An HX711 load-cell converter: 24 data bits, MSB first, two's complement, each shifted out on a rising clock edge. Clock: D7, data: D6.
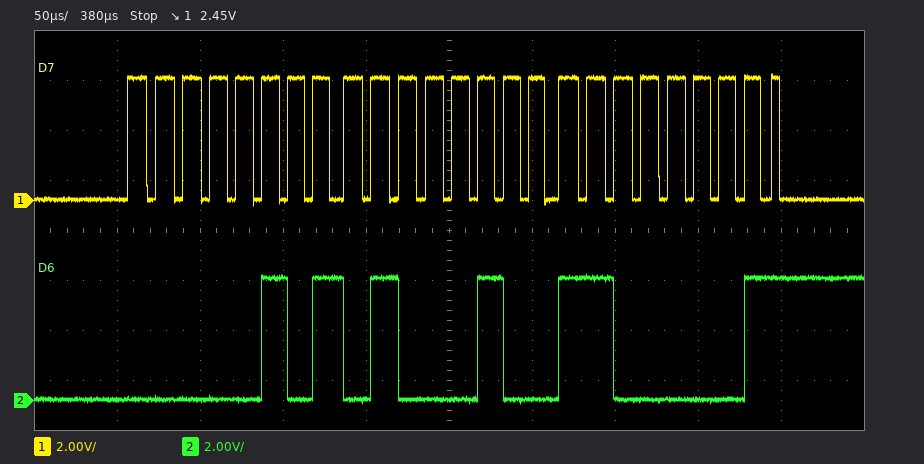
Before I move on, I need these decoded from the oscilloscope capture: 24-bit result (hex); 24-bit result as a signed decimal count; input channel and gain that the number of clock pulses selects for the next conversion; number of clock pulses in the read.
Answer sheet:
0x0544C1
345281
channel A, gain 128
25
